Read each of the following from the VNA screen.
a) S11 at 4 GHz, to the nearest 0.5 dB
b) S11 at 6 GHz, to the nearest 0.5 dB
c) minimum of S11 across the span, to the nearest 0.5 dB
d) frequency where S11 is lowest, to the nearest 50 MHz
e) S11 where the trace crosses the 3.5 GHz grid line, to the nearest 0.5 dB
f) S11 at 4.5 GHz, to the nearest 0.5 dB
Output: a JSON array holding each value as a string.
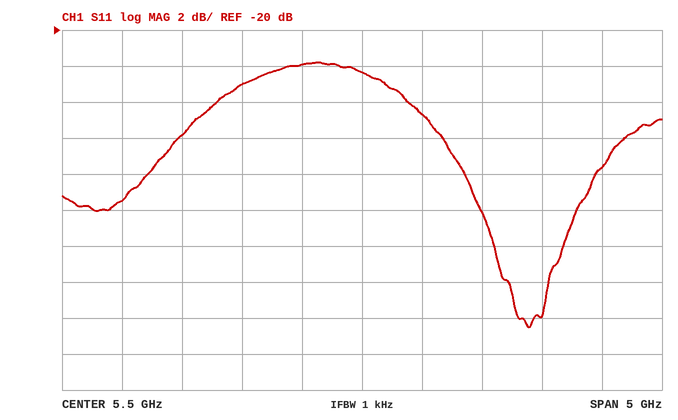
["-26.0 dB", "-24.5 dB", "-36.5 dB", "6.90 GHz", "-29.5 dB", "-23.0 dB"]
